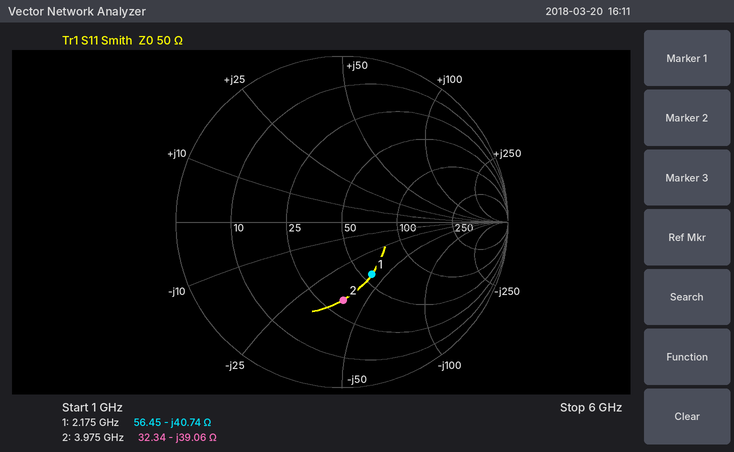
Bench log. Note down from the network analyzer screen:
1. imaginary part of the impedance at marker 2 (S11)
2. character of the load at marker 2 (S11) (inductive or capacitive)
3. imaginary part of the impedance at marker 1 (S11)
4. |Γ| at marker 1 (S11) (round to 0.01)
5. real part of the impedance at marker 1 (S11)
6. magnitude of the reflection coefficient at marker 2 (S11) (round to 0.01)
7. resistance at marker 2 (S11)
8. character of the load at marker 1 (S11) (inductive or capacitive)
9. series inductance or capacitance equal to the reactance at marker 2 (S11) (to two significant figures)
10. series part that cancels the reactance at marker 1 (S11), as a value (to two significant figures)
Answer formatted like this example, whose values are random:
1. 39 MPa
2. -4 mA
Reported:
1. -39.06 Ω
2. capacitive
3. -40.74 Ω
4. 0.36
5. 56.45 Ω
6. 0.47
7. 32.34 Ω
8. capacitive
9. 1.0 pF
10. 3.0 nH
